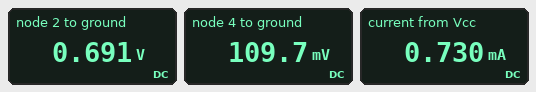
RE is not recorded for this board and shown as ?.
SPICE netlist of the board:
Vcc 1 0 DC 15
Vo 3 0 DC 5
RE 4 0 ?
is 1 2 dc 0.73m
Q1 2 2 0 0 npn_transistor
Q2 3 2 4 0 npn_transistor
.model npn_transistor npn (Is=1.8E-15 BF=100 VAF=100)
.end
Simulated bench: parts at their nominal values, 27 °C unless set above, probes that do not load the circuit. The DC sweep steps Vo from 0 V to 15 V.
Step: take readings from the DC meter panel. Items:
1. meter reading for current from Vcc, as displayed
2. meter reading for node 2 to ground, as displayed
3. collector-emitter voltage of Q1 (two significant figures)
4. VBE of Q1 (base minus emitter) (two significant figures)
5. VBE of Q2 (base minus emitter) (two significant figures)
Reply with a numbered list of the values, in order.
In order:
1. 0.730 mA
2. 0.691 V
3. 690 mV
4. 690 mV
5. 580 mV
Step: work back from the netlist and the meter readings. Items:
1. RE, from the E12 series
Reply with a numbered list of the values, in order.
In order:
1. 10 kΩ
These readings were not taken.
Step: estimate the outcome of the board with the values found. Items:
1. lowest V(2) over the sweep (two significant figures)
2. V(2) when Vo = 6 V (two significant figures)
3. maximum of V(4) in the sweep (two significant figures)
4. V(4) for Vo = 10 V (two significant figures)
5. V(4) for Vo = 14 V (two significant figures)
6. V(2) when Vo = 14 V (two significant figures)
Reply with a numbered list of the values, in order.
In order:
1. 670 mV
2. 690 mV
3. 110 mV
4. 110 mV
5. 110 mV
6. 690 mV
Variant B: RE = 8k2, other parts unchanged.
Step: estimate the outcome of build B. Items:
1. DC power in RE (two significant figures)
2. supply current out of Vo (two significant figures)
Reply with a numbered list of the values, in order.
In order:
1. 1.4 µW
2. 13 µA
